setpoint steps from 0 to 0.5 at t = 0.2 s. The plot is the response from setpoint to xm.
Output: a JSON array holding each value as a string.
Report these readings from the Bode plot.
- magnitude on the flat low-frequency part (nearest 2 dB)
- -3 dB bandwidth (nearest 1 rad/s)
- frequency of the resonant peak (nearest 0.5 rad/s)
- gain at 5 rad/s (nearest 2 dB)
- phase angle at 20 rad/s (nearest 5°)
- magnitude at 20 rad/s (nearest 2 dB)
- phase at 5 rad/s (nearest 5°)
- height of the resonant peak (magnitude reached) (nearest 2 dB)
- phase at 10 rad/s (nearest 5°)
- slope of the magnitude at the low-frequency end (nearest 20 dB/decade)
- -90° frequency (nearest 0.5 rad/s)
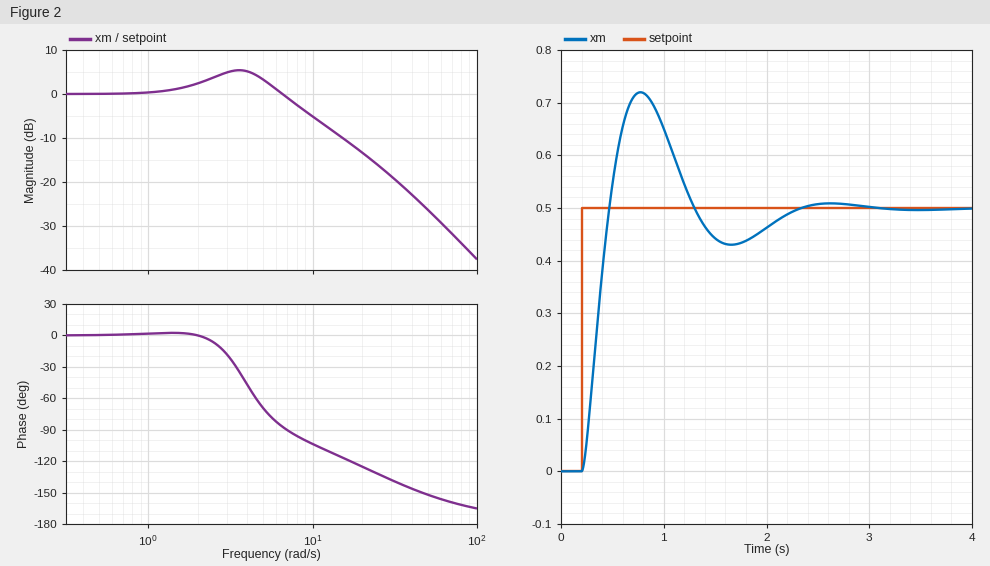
["0 dB", "8 rad/s", "3.5 rad/s", "4 dB", "-125°", "-14 dB", "-70°", "6 dB", "-105°", "0 dB/decade", "7.0 rad/s"]
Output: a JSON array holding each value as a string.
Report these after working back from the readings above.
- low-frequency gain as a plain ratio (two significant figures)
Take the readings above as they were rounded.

["1.0"]
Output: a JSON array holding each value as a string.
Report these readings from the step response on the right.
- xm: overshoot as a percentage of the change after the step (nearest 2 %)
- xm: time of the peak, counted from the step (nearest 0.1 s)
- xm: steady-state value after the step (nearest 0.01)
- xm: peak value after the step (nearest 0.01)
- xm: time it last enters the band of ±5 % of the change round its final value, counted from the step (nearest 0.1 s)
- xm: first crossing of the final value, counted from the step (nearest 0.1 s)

["44 %", "0.6 s", "0.50", "0.72", "1.9 s", "0.3 s"]
